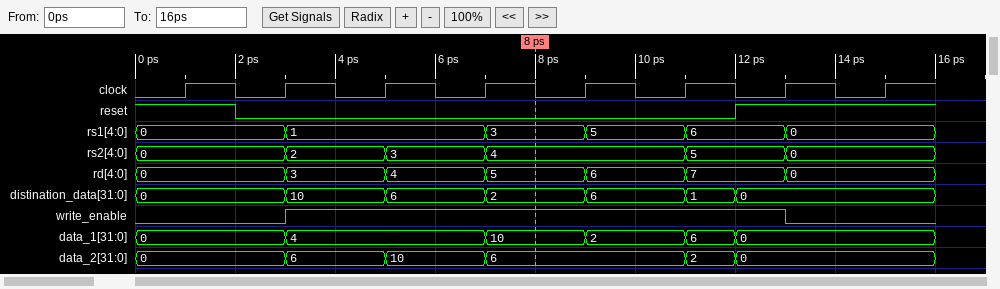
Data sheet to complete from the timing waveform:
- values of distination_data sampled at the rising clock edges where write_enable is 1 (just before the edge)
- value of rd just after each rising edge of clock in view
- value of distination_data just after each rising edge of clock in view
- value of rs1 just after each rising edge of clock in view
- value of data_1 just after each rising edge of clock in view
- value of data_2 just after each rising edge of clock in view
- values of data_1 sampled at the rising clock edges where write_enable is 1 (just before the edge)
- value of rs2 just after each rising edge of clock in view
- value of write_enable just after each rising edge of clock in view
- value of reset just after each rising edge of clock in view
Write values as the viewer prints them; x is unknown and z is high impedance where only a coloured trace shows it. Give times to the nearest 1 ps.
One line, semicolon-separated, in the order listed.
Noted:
10, 6, 2, 6, 0; 0, 3, 4, 5, 6, 7, 0, 0; 0, 10, 6, 2, 6, 1, 0, 0; 0, 1, 1, 3, 5, 6, 0, 0; 0, 4, 4, 10, 2, 6, 0, 0; 0, 6, 10, 6, 6, 2, 0, 0; 4, 4, 10, 2, 0; 0, 2, 3, 4, 4, 5, 0, 0; 0 1 1 1 1 1 0 0; 1 0 0 0 0 0 1 1
